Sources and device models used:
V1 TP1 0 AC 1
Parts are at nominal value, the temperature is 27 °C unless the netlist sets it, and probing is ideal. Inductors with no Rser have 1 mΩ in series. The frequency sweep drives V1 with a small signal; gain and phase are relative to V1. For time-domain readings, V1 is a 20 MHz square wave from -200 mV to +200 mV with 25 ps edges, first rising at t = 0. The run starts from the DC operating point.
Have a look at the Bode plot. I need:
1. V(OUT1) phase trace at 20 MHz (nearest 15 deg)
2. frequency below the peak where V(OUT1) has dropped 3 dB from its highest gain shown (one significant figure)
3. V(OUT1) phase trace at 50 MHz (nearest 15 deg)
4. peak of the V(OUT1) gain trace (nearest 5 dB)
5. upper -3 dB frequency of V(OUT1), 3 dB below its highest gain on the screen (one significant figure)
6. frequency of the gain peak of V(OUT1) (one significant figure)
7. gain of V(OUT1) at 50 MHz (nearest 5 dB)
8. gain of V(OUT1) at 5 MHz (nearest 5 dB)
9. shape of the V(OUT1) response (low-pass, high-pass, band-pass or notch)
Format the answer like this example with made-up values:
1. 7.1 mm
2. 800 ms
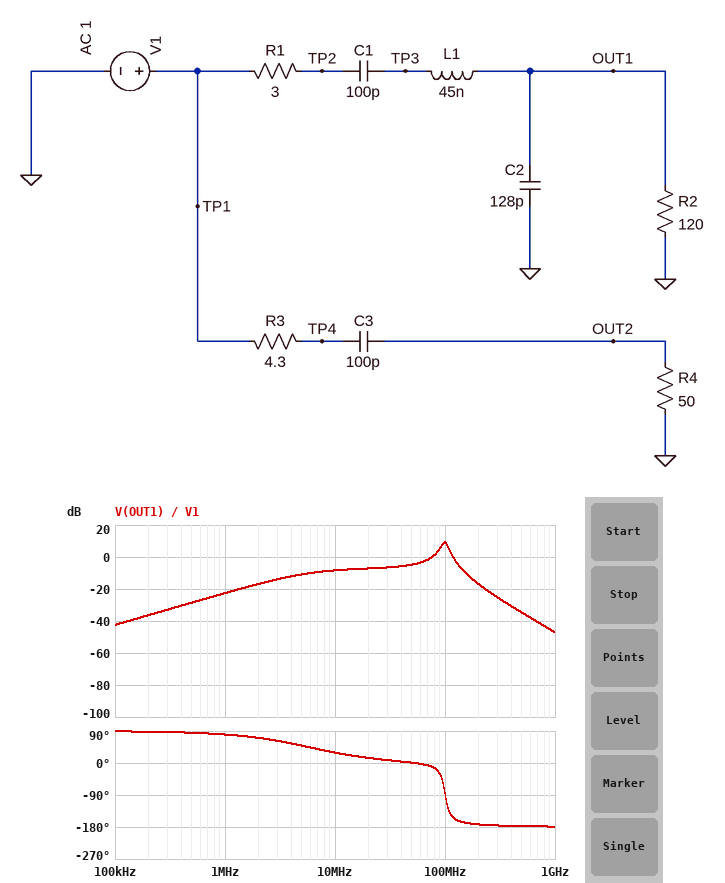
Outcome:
1. 15 deg
2. 90 MHz
3. 0 deg
4. 10 dB
5. 100 MHz
6. 100 MHz
7. -5 dB
8. -10 dB
9. band-pass
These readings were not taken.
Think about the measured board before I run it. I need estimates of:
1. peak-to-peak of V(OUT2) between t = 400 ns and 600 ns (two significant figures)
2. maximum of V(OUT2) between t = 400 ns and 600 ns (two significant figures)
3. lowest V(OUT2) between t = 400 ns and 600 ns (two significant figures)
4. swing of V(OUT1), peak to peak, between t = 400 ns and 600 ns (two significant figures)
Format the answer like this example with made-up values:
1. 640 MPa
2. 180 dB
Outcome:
1. 730 mV
2. 360 mV
3. -360 mV
4. 610 mV
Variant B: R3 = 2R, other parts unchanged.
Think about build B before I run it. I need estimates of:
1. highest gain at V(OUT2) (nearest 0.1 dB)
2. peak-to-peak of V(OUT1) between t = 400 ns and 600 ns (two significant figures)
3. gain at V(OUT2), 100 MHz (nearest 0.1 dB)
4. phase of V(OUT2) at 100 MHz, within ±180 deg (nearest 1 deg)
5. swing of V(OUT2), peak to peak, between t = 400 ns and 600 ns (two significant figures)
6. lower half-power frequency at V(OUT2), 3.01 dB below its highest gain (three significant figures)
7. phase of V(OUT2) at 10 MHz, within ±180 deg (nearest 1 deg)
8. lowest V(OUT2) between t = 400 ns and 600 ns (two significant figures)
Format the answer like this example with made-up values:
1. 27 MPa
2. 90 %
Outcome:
1. -0.3 dB
2. 610 mV
3. -0.7 dB
4. 17 deg
5. 760 mV
6. 30.6 MHz
7. 72 deg
8. -380 mV
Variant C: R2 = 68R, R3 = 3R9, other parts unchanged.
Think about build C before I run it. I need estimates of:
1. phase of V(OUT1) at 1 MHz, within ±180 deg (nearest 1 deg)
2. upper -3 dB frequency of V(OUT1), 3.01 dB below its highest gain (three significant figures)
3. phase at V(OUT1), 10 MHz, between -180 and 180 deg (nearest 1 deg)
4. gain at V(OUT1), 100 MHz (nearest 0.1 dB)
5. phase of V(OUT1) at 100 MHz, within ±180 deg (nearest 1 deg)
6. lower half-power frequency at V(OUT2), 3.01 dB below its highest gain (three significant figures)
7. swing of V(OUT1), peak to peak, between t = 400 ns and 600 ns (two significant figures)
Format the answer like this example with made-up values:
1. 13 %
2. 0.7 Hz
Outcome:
1. 84 deg
2. 108 MHz
3. 45 deg
4. 7.4 dB
5. -83 deg
6. 29.5 MHz
7. 560 mV
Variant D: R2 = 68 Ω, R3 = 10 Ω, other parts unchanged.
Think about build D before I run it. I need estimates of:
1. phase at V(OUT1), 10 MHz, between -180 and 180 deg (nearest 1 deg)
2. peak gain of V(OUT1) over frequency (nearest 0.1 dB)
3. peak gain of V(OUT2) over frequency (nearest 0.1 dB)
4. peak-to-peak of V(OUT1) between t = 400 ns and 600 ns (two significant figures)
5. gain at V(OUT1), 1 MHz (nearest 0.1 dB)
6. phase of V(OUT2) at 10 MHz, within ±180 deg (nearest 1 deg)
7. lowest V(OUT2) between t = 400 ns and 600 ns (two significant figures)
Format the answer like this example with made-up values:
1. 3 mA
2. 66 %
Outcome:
1. 45 deg
2. 7.4 dB
3. -1.6 dB
4. 560 mV
5. -27.4 dB
6. 69 deg
7. -330 mV
